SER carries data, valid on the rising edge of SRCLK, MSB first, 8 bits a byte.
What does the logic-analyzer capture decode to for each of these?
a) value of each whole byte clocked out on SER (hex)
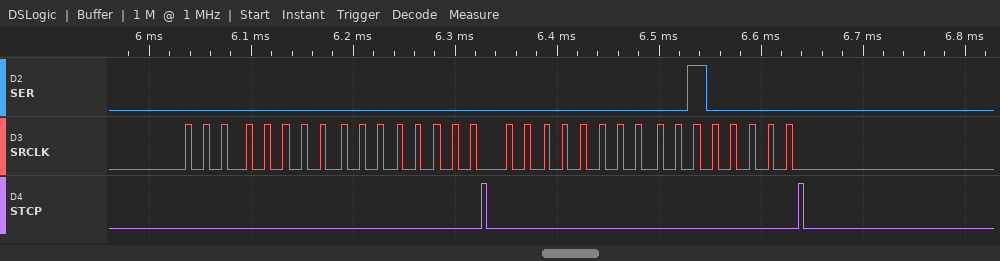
0x00 0x00 0x00 0x20
